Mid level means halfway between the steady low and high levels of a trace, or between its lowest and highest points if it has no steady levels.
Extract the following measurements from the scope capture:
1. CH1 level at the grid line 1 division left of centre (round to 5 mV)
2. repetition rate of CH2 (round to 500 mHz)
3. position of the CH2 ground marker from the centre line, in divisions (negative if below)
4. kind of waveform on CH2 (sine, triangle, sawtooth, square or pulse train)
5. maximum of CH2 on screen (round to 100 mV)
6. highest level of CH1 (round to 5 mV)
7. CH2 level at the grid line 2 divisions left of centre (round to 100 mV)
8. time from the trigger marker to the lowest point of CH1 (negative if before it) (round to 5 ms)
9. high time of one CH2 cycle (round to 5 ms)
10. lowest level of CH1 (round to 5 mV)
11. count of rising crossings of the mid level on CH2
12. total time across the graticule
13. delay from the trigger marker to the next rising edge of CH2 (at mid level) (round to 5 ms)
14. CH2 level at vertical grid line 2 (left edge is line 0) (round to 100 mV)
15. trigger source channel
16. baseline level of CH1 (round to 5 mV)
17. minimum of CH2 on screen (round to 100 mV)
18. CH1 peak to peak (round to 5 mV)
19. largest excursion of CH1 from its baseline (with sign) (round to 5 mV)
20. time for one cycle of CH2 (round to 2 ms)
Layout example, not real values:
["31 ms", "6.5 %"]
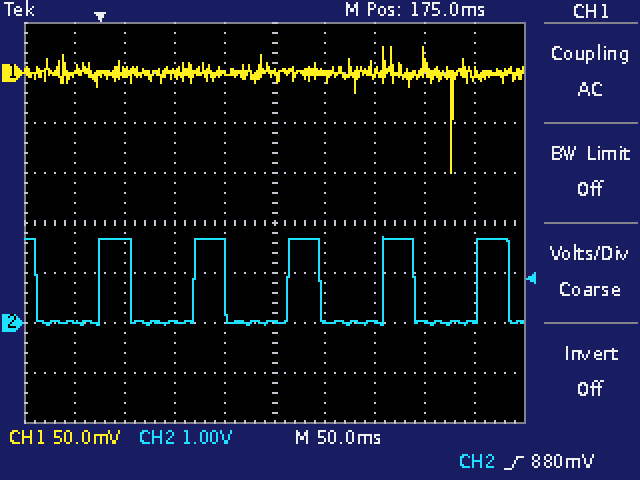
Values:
["0 mV", "10.5 Hz", "-2.0 div", "pulse train", "1.7 V", "25 mV", "0.0 V", "+350 ms", "30 ms", "-100 mV", "5", "500 ms", "95 ms", "1.7 V", "CH2", "0 mV", "0.0 V", "125 mV", "-100 mV", "94 ms"]
